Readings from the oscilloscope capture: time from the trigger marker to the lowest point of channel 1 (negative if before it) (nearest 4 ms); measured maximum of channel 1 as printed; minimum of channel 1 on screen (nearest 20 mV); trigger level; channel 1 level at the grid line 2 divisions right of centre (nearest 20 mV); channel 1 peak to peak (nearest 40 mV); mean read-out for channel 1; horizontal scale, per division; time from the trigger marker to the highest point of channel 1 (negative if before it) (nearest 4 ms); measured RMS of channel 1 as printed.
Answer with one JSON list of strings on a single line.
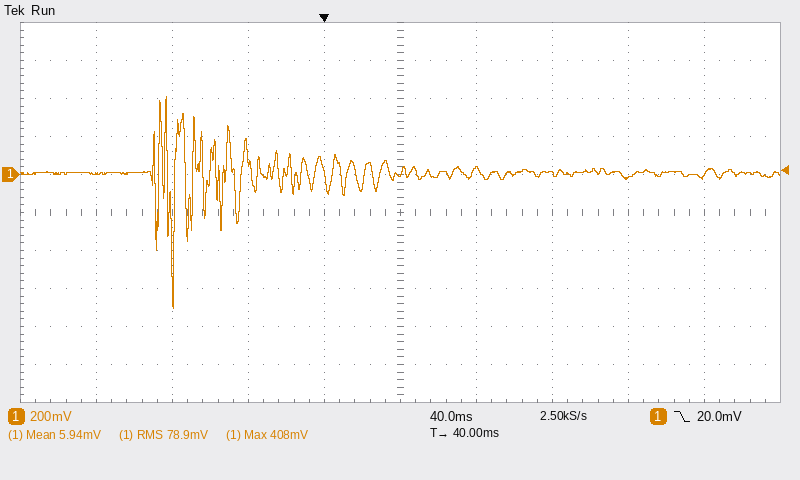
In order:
["-80 ms", "408 mV", "-700 mV", "20.0 mV", "0 mV", "1.12 V", "5.94 mV", "40 ms", "-84 ms", "78.9 mV"]
